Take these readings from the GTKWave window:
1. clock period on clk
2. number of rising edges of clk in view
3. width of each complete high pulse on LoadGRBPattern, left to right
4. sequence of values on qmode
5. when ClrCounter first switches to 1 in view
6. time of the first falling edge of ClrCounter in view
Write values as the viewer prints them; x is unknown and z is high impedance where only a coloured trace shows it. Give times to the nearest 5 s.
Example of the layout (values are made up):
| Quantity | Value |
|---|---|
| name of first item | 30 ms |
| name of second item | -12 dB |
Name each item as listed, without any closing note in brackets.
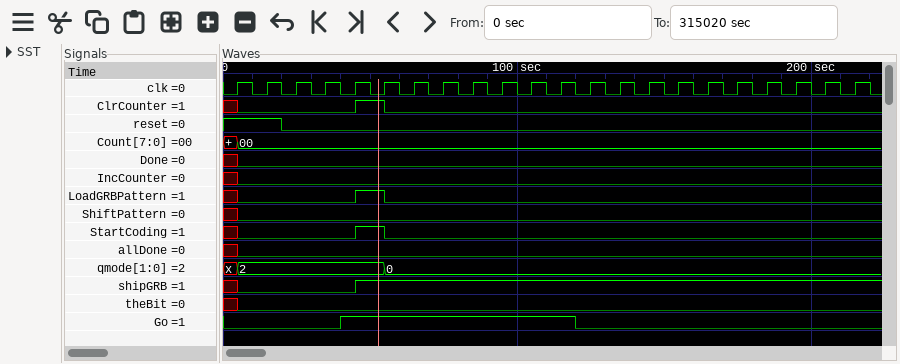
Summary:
| Quantity | Value |
|---|---|
| clock period on clk | 10 s |
| number of rising edges of clk in view | 22 |
| width of each complete high pulse on LoadGRBPattern, left to right | 10 s |
| sequence of values on qmode | x, 2, 0 |
| when ClrCounter first switches to 1 in view | 45 s |
| time of the first falling edge of ClrCounter in view | 55 s |
